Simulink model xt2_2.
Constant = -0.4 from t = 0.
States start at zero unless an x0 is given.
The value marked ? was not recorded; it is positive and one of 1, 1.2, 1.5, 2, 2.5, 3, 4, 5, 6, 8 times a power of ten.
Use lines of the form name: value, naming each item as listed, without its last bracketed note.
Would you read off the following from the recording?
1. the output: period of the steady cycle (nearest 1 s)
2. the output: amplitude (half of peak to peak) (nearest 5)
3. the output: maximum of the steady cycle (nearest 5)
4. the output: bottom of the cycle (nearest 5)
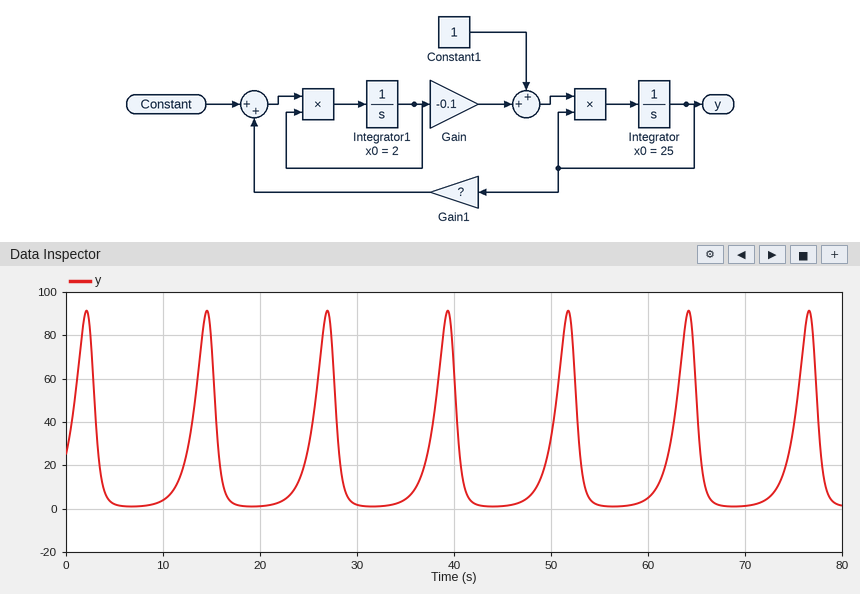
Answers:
the output: period of the steady cycle: 12 s
the output: amplitude (half of peak to peak): 45
the output: maximum of the steady cycle: 90
the output: bottom of the cycle: 0
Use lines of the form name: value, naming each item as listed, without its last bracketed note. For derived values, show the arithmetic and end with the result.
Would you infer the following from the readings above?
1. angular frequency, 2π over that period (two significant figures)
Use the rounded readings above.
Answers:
angular frequency, 2π over that period: 2π / 12 = 0.52 rad/s
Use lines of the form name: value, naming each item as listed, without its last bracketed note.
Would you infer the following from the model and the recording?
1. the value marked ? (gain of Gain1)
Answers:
the value marked ?: 0.02
